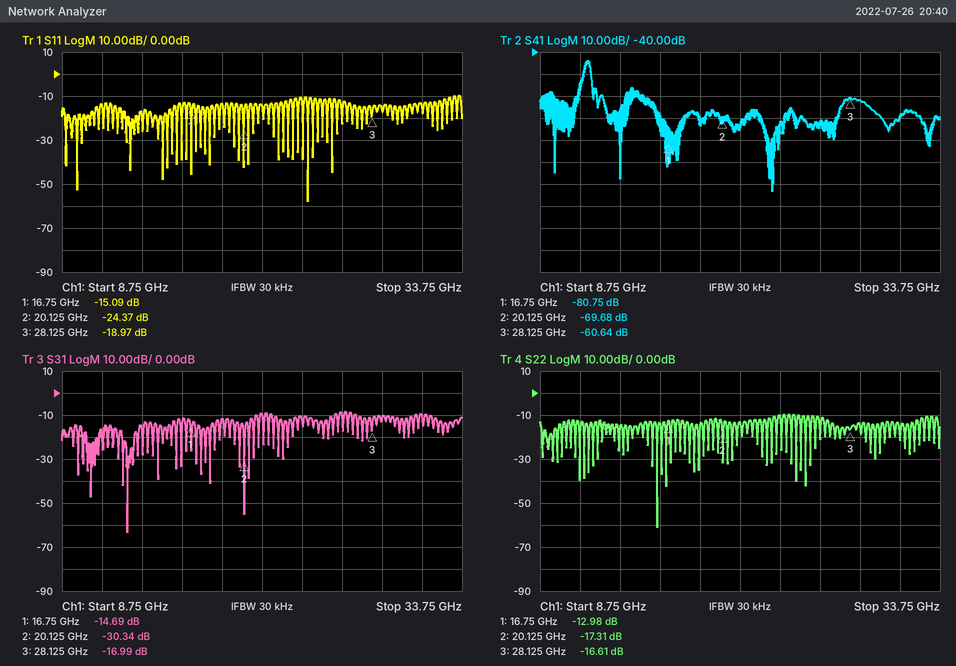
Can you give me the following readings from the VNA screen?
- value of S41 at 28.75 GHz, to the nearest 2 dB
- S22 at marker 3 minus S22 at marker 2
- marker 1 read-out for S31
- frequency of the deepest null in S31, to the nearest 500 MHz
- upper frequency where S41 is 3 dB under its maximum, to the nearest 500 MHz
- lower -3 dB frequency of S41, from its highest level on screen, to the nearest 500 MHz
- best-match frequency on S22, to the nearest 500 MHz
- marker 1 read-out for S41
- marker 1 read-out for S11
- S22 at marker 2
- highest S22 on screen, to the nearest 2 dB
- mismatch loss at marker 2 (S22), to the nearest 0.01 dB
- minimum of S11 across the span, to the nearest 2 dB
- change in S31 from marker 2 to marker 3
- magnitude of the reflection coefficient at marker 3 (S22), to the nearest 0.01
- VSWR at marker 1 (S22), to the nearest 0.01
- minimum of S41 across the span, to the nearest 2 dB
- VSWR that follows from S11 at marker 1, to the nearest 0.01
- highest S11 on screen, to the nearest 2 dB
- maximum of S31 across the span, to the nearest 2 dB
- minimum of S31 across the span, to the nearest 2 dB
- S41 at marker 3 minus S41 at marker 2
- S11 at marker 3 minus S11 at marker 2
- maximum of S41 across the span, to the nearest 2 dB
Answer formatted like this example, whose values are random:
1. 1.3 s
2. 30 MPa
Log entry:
1. -62 dB
2. 0.70 dB
3. -14.69 dB
4. 13.0 GHz
5. 12.0 GHz
6. 11.5 GHz
7. 16.0 GHz
8. -80.75 dB
9. -15.09 dB
10. -17.31 dB
11. -10 dB
12. 0.08 dB
13. -58 dB
14. 13.35 dB
15. 0.15
16. 1.58
17. -104 dB
18. 1.43
19. -10 dB
20. -8 dB
21. -64 dB
22. 9.04 dB
23. 5.40 dB
24. -44 dB
